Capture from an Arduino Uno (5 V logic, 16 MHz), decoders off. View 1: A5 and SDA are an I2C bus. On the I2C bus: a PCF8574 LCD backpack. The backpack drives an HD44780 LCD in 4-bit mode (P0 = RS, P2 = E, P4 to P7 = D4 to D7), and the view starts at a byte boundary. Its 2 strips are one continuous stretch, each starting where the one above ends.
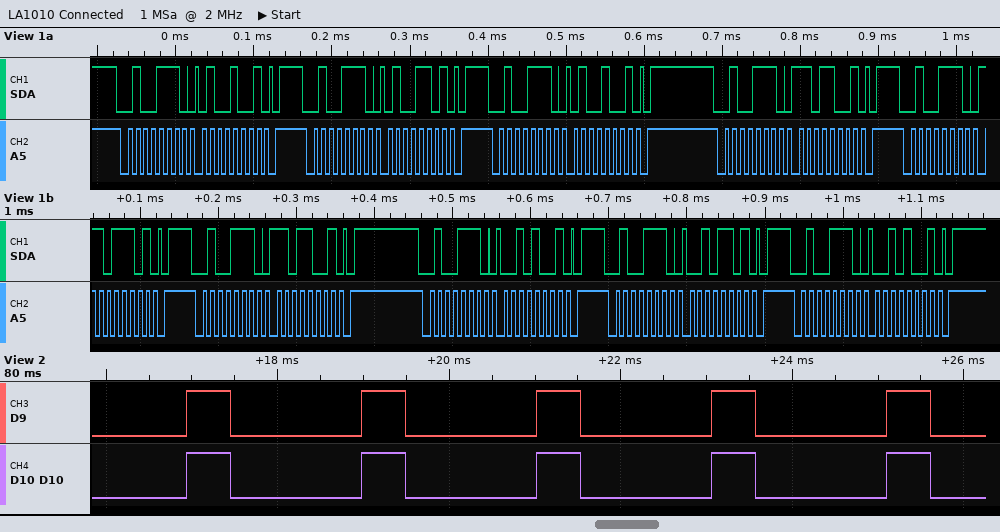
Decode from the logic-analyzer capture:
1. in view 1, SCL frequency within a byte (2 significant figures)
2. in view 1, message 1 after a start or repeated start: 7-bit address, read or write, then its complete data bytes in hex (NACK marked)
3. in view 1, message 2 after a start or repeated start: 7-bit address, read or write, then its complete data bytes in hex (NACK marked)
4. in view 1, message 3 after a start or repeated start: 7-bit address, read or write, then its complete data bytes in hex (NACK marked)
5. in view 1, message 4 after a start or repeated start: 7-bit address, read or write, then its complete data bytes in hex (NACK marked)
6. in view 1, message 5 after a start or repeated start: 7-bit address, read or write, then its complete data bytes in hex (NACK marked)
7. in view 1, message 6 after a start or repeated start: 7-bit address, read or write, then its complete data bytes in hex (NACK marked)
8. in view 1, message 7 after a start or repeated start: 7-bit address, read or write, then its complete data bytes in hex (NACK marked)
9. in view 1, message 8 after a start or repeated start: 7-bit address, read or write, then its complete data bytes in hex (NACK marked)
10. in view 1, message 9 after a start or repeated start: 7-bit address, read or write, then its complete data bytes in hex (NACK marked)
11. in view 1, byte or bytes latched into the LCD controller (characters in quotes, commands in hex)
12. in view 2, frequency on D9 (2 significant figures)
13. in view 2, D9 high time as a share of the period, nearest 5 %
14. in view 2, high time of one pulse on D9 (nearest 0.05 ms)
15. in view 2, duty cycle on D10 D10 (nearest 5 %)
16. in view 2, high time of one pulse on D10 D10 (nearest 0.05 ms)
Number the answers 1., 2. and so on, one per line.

1. 100 kHz
2. 0x27 write: 49
3. 0x27 write: 4D
4. 0x27 write: 49
5. 0x27 write: D9
6. 0x27 write: DD
7. 0x27 write: D9
8. 0x27 write: 29
9. 0x27 write: 2D
10. 0x27 write: 29
11. 'M'
12. 490 Hz
13. 25 %
14. 0.50 ms
15. 25 %
16. 0.50 ms
